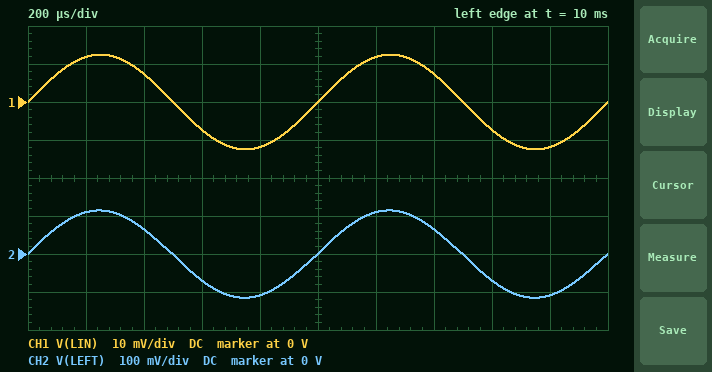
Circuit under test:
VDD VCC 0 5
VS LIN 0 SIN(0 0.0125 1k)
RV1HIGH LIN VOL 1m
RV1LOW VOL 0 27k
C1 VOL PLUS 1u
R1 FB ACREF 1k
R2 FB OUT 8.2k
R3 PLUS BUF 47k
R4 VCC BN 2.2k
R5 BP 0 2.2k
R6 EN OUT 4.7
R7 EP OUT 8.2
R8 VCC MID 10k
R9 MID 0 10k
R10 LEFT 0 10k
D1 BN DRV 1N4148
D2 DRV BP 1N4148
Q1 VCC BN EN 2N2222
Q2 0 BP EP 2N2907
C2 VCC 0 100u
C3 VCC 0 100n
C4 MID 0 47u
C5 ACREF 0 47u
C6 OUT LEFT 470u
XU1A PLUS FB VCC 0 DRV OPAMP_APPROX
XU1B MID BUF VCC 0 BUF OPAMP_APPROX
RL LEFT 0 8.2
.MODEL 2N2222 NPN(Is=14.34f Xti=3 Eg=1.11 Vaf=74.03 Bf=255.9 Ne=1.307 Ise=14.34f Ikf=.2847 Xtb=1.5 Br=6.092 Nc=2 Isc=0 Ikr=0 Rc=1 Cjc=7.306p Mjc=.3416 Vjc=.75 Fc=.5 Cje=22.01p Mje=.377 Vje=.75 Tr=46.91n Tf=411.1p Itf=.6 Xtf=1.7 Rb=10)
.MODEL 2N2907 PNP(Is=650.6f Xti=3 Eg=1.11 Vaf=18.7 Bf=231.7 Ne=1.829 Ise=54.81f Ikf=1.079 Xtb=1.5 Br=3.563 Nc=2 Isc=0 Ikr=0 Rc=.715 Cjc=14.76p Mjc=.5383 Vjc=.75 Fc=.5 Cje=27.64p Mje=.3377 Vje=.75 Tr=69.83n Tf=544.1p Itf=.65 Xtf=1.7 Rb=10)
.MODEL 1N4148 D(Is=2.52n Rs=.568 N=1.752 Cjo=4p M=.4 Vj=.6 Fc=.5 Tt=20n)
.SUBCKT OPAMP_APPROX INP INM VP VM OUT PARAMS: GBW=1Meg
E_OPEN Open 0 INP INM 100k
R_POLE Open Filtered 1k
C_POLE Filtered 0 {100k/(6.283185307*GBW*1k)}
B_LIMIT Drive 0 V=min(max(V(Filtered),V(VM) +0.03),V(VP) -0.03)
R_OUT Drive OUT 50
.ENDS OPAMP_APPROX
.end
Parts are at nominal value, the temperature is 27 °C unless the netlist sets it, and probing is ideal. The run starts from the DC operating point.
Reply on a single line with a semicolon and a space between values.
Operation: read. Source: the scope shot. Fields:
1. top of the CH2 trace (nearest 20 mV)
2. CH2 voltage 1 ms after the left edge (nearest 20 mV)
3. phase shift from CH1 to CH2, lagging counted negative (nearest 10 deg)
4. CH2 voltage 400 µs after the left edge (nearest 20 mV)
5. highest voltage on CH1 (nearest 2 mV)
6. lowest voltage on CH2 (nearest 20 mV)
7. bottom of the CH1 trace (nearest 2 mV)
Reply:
120 mV; 0 V; 0 deg; 60 mV; 12 mV; -120 mV; -12 mV
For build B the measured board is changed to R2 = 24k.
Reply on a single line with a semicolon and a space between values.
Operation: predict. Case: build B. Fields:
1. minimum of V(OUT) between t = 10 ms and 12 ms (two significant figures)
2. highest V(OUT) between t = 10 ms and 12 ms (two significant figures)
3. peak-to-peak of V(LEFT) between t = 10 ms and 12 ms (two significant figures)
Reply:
2.2 V; 2.8 V; 620 mV
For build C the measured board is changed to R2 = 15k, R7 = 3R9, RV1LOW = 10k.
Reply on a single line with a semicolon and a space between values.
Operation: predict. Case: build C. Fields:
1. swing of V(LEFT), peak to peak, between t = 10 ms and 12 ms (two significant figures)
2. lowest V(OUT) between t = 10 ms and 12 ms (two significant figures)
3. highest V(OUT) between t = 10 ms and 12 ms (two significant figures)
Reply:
400 mV; 2.3 V; 2.7 V
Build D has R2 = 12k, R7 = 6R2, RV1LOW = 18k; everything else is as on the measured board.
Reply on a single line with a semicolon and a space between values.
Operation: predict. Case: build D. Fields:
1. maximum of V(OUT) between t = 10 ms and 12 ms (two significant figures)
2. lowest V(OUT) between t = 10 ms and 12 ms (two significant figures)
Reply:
2.7 V; 2.3 V
